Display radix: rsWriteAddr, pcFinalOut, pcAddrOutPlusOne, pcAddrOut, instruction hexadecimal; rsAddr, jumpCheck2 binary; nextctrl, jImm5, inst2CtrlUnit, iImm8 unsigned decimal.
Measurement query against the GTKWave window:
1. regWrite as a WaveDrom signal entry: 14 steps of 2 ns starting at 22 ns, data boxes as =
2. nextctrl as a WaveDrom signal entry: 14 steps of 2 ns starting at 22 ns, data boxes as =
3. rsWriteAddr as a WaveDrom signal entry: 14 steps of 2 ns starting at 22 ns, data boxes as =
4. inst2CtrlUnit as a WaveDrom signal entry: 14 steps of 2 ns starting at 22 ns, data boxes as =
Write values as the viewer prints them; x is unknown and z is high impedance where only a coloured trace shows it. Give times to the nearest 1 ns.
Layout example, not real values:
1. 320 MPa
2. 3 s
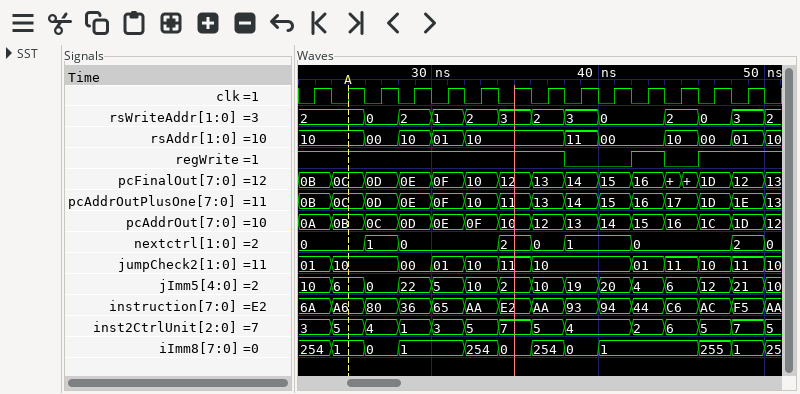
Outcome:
1. {name: 'regWrite', wave: '1.......0.101.'}
2. {name: 'nextctrl', wave: '=.==..===.=..=', data: '0 1 0 2 0 1 0 2'}
3. {name: 'rsWriteAddr', wave: '=.========.===', data: '2 0 2 1 2 3 2 3 0 2 0 3'}
4. {name: 'inst2CtrlUnit', wave: '=========.====', data: '3 5 4 1 3 5 7 5 4 2 6 5 7'}
